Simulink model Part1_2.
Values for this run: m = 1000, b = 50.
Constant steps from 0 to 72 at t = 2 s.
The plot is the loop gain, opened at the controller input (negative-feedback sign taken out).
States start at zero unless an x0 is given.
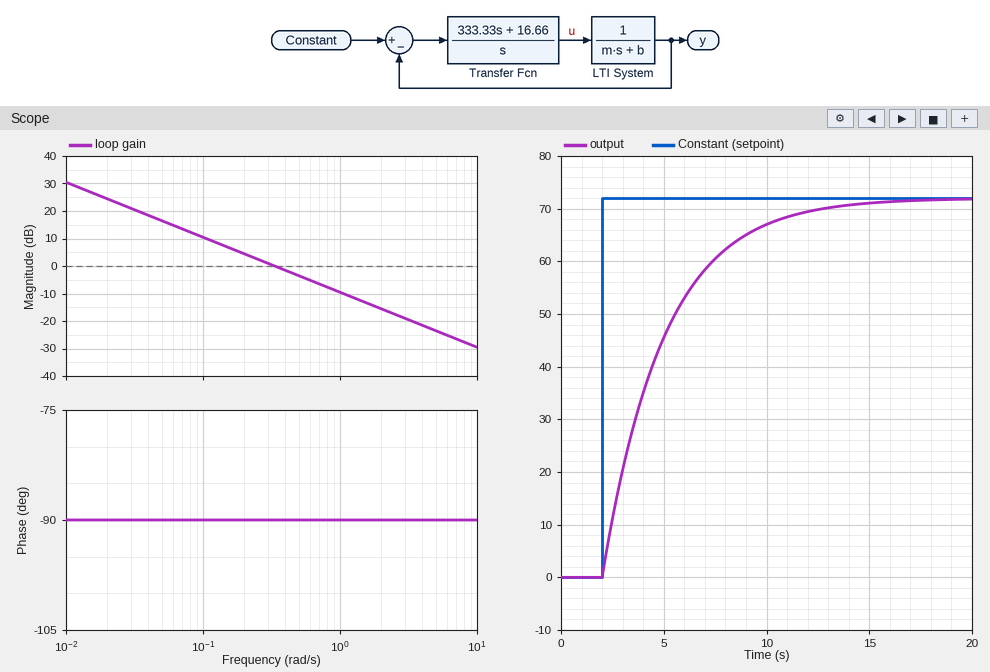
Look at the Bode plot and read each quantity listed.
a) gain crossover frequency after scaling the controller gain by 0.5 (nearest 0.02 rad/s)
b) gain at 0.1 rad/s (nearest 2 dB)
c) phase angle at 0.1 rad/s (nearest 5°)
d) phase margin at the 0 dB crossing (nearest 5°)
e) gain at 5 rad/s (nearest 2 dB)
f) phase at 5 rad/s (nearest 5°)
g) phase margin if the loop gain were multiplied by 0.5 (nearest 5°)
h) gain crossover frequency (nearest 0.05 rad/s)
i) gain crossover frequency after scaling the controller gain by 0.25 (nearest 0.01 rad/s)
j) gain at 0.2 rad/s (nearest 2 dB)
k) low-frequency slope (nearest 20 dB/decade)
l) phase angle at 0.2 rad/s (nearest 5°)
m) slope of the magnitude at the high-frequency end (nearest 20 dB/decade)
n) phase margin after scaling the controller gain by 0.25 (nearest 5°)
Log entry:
0.16 rad/s
10 dB
-90°
90°
-24 dB
-90°
90°
0.35 rad/s
0.08 rad/s
4 dB
-20 dB/decade
-90°
-20 dB/decade
90°
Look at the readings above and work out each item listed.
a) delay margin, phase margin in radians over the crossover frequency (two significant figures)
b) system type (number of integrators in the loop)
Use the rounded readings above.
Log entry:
4.5 s
1
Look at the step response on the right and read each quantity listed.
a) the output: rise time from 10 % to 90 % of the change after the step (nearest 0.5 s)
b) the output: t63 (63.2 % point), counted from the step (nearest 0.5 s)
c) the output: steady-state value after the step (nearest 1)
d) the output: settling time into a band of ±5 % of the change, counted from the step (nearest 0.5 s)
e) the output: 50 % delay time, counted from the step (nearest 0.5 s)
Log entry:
6.5 s
3.0 s
72
9.0 s
2.0 s
